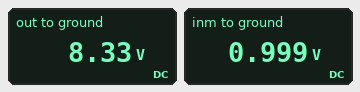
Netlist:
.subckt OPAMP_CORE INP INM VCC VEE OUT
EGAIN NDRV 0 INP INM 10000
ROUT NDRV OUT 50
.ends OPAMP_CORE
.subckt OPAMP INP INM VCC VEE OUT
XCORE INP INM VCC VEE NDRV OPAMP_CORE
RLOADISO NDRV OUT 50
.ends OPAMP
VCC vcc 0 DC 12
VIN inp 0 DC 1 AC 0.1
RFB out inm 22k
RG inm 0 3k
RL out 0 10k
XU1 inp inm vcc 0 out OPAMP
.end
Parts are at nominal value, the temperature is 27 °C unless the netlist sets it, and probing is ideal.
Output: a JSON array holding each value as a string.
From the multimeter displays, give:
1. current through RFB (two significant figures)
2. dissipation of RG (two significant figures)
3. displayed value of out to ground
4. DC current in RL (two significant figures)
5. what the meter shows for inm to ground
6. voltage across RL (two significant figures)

["330 µA", "330 µW", "8.33 V", "830 µA", "0.999 V", "8.3 V"]
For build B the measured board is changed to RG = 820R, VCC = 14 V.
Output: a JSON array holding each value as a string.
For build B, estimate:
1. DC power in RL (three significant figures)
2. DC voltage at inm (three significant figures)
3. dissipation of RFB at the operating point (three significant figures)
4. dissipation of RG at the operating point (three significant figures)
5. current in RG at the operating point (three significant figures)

["77.0 mW", "997 mV", "32.5 mW", "1.21 mW", "1.22 mA"]
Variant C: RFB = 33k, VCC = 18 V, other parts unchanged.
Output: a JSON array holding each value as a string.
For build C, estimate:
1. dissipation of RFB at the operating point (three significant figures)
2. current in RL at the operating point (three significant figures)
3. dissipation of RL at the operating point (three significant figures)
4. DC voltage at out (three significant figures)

["3.66 mW", "1.20 mA", "14.4 mW", "12.0 V"]
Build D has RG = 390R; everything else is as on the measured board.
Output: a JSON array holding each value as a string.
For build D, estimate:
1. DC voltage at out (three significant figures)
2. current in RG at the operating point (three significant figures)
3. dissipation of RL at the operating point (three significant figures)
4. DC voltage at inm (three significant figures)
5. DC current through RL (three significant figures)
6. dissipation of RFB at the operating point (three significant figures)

["57.1 V", "2.55 mA", "326 mW", "994 mV", "5.71 mA", "143 mW"]
